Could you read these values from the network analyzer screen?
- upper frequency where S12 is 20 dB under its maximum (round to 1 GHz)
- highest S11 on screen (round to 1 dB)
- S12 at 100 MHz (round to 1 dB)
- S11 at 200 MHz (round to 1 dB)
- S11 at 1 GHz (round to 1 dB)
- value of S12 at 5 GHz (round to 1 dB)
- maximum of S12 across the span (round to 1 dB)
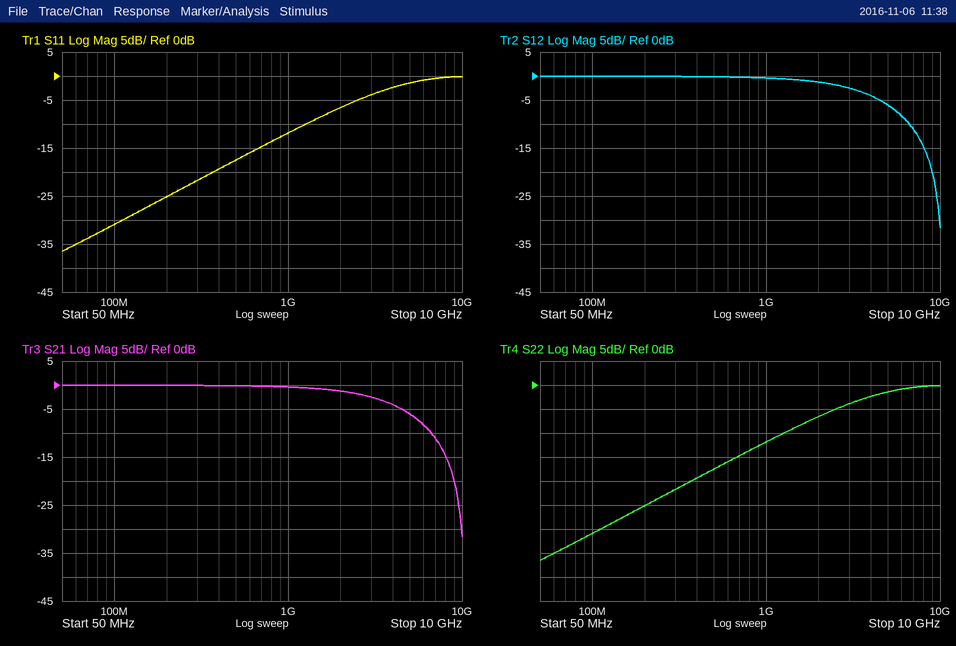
9 GHz
0 dB
0 dB
-25 dB
-12 dB
-6 dB
0 dB
